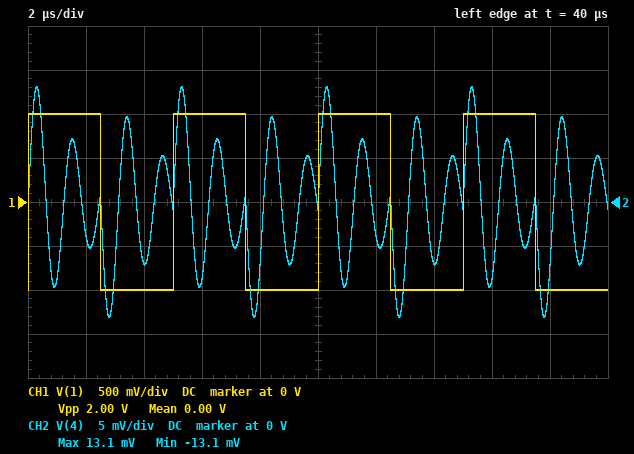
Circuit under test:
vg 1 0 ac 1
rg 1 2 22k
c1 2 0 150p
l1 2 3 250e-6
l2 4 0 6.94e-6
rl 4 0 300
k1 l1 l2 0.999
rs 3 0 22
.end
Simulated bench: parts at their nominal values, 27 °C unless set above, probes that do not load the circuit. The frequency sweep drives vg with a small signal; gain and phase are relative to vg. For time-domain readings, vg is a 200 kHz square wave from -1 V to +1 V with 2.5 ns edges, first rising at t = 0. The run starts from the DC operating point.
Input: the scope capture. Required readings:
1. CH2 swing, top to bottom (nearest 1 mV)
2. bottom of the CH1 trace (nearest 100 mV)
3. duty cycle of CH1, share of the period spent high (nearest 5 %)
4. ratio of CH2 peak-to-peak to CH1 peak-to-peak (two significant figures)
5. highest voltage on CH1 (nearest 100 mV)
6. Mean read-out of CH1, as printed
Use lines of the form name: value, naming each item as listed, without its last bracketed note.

CH2 swing, top to bottom: 26 mV
bottom of the CH1 trace: -1.0 V
duty cycle of CH1, share of the period spent high: 50 %
ratio of CH2 peak-to-peak to CH1 peak-to-peak: 0.013
highest voltage on CH1: 1.0 V
Mean read-out of CH1, as printed: 0.00 V
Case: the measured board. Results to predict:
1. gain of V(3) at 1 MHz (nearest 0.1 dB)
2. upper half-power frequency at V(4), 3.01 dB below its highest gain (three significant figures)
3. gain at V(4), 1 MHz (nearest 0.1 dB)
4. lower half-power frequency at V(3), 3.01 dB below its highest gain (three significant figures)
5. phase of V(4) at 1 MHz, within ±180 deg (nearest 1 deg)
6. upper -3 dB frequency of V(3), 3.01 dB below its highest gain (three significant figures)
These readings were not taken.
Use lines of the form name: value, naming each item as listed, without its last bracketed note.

gain of V(3) at 1 MHz: -54.5 dB
upper half-power frequency at V(4), 3.01 dB below its highest gain: 905 kHz
gain at V(4), 1 MHz: -33.1 dB
lower half-power frequency at V(3), 3.01 dB below its highest gain: 729 kHz
phase of V(4) at 1 MHz, within ±180 deg: -64 deg
upper -3 dB frequency of V(3), 3.01 dB below its highest gain: 891 kHz
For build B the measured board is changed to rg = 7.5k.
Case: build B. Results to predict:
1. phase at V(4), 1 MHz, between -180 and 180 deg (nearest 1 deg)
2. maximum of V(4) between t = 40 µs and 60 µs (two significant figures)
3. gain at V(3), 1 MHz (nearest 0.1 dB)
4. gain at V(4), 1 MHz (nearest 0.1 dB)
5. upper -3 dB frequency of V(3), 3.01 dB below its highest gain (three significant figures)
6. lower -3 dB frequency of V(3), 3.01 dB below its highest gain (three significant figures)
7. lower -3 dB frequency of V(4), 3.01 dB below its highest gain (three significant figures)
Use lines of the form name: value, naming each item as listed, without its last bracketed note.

phase at V(4), 1 MHz, between -180 and 180 deg: -52 deg
maximum of V(4) between t = 40 µs and 60 µs: 40 mV
gain at V(3), 1 MHz: -46.3 dB
gain at V(4), 1 MHz: -24.9 dB
upper -3 dB frequency of V(3), 3.01 dB below its highest gain: 922 kHz
lower -3 dB frequency of V(3), 3.01 dB below its highest gain: 663 kHz
lower -3 dB frequency of V(4), 3.01 dB below its highest gain: 705 kHz
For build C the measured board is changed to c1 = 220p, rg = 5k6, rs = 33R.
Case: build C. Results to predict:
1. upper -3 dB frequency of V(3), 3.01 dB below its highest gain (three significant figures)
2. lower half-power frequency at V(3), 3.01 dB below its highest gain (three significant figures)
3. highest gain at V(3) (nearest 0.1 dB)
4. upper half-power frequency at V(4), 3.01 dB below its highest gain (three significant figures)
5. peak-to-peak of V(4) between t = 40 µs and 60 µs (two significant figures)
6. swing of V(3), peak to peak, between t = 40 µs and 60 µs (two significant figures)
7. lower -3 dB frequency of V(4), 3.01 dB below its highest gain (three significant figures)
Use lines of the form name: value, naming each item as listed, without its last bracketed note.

upper -3 dB frequency of V(3), 3.01 dB below its highest gain: 764 kHz
lower half-power frequency at V(3), 3.01 dB below its highest gain: 542 kHz
highest gain at V(3): -34.6 dB
upper half-power frequency at V(4), 3.01 dB below its highest gain: 797 kHz
peak-to-peak of V(4) between t = 40 µs and 60 µs: 110 mV
swing of V(3), peak to peak, between t = 40 µs and 60 µs: 27 mV
lower -3 dB frequency of V(4), 3.01 dB below its highest gain: 580 kHz
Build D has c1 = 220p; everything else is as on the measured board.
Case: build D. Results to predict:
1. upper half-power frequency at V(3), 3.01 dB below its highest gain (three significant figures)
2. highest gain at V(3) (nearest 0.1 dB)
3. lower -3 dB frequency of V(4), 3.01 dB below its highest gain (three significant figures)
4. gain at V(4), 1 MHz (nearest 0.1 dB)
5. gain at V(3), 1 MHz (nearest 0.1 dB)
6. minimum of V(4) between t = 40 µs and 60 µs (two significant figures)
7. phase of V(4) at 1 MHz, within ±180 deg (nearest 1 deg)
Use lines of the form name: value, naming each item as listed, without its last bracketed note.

upper half-power frequency at V(3), 3.01 dB below its highest gain: 728 kHz
highest gain at V(3): -44.4 dB
lower -3 dB frequency of V(4), 3.01 dB below its highest gain: 624 kHz
gain at V(4), 1 MHz: -40.1 dB
gain at V(3), 1 MHz: -61.5 dB
minimum of V(4) between t = 40 µs and 60 µs: -16 mV
phase of V(4) at 1 MHz, within ±180 deg: -78 deg
